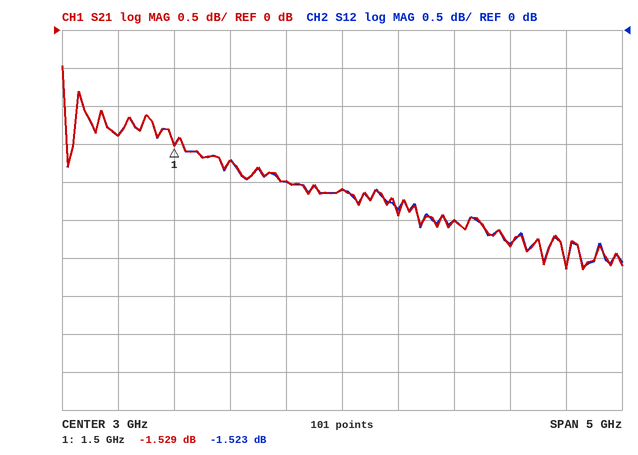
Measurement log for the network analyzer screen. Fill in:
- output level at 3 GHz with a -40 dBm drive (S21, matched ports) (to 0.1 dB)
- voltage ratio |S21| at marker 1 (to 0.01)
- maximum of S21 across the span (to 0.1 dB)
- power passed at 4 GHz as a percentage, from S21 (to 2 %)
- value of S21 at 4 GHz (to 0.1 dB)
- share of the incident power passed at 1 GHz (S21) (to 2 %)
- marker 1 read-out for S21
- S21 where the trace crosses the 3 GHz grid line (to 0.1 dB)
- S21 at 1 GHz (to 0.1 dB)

-42.1 dBm
0.84
-0.5 dB
56 %
-2.5 dB
72 %
-1.529 dB
-2.1 dB
-1.4 dB
